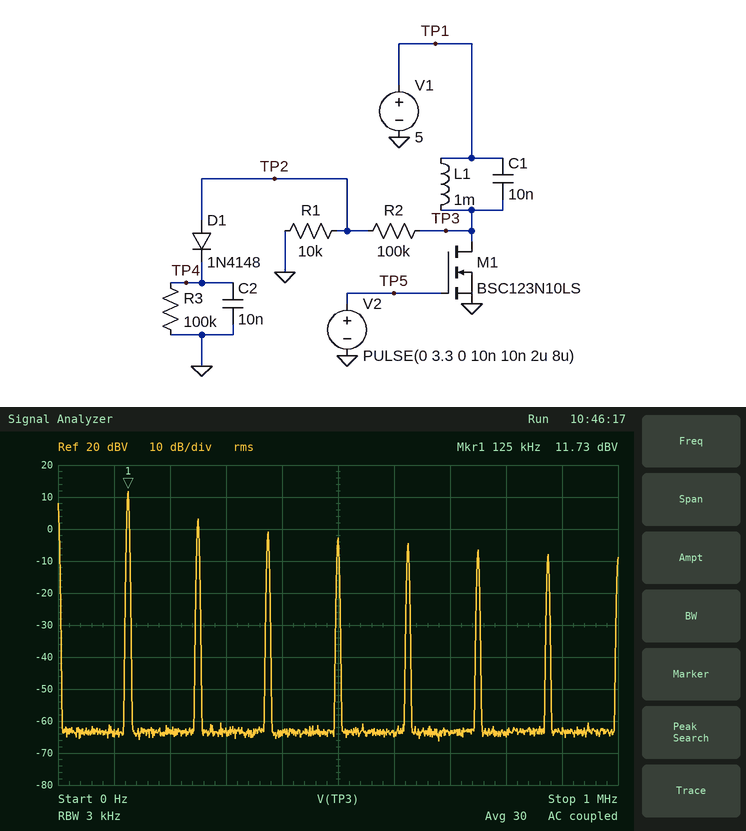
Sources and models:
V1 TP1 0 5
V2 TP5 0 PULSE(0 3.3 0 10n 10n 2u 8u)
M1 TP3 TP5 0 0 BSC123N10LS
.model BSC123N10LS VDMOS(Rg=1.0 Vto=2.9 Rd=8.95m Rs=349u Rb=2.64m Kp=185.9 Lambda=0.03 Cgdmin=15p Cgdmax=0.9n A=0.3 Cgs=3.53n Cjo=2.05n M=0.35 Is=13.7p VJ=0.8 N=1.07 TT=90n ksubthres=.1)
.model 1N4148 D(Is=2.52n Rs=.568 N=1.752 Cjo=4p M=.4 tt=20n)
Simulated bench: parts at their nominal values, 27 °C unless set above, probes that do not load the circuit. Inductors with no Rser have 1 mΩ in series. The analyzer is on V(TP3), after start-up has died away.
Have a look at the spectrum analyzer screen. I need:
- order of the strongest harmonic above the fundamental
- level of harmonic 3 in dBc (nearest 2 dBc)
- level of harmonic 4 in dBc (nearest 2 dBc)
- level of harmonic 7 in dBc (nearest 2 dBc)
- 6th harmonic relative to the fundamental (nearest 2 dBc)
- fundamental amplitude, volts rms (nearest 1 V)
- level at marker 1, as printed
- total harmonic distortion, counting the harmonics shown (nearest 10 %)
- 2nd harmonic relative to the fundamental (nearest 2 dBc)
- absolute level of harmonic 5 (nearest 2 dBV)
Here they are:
2
-12 dBc
-14 dBc
-20 dBc
-18 dBc
4 V
11.73 dBV
50 %
-8 dBc
-4 dBV
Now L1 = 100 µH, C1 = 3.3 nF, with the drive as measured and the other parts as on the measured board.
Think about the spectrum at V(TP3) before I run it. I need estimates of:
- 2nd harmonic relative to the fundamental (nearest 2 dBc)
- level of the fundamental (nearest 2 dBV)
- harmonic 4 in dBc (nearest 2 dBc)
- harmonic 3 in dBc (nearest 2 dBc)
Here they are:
-2 dBc
16 dBV
-12 dBc
-6 dBc
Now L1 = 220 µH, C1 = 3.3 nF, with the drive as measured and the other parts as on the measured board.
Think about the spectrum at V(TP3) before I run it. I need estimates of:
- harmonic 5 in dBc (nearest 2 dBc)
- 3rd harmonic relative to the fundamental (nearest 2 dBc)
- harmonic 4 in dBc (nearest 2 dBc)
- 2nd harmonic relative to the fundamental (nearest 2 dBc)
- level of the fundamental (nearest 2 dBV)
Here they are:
-42 dBc
-26 dBc
-24 dBc
-6 dBc
16 dBV
